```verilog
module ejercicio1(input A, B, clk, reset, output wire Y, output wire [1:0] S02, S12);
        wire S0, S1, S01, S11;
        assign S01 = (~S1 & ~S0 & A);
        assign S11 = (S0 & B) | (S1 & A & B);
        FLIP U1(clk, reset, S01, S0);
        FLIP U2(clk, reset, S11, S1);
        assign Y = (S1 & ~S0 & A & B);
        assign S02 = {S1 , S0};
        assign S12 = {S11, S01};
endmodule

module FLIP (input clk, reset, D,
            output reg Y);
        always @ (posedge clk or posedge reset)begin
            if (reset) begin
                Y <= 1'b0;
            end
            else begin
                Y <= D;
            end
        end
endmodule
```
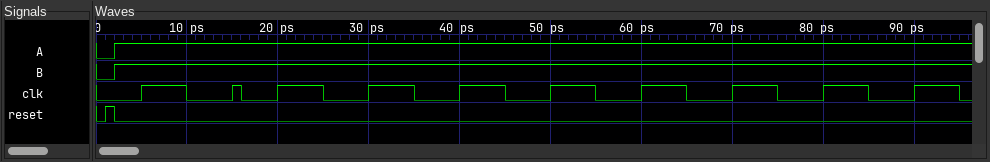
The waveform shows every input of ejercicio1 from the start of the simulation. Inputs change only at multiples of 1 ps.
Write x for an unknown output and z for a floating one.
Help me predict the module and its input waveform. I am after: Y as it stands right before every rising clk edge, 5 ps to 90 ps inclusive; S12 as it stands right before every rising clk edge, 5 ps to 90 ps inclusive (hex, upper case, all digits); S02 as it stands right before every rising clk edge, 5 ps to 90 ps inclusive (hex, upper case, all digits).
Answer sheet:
0 0 1 1 1 1 1 1 1 1
1, 2, 2, 2, 2, 2, 2, 2, 2, 2
0, 1, 2, 2, 2, 2, 2, 2, 2, 2
